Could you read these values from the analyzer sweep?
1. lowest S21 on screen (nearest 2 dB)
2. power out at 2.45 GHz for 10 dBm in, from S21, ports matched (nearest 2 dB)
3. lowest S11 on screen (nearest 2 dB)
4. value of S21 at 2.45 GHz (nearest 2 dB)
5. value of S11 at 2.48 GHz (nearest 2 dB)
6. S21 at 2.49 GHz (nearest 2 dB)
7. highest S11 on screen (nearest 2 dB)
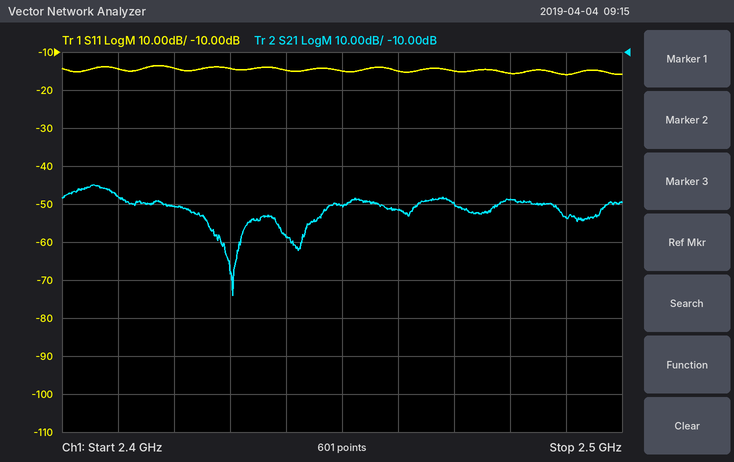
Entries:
-74 dB
-40 dBm
-16 dB
-50 dB
-16 dB
-54 dB
-14 dB
